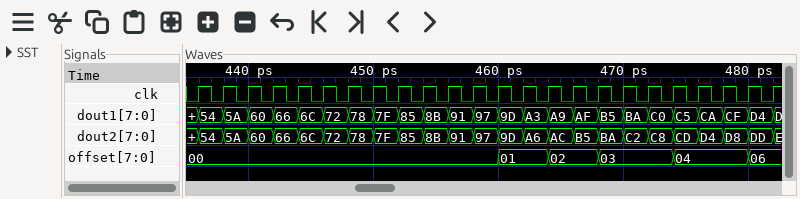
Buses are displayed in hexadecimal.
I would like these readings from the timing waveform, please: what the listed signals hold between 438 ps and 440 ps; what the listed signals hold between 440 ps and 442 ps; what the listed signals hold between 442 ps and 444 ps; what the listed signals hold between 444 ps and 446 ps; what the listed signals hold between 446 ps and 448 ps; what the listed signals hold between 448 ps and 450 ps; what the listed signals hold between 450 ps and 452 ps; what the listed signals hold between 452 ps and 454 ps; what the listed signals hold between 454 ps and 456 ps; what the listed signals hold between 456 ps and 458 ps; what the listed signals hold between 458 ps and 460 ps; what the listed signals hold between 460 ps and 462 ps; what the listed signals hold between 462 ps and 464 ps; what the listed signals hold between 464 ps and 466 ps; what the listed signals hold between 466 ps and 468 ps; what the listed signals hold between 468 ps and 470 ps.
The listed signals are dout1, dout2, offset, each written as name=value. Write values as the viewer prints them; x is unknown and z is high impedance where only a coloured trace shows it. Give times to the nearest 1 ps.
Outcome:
dout1=5A, dout2=5A, offset=00
dout1=60, dout2=60, offset=00
dout1=66, dout2=66, offset=00
dout1=6C, dout2=6C, offset=00
dout1=72, dout2=72, offset=00
dout1=78, dout2=78, offset=00
dout1=7F, dout2=7F, offset=00
dout1=85, dout2=85, offset=00
dout1=8B, dout2=8B, offset=00
dout1=91, dout2=91, offset=00
dout1=97, dout2=97, offset=00
dout1=9D, dout2=9D, offset=01
dout1=A3, dout2=A6, offset=01
dout1=A9, dout2=AC, offset=02
dout1=AF, dout2=B5, offset=02
dout1=B5, dout2=BA, offset=03
